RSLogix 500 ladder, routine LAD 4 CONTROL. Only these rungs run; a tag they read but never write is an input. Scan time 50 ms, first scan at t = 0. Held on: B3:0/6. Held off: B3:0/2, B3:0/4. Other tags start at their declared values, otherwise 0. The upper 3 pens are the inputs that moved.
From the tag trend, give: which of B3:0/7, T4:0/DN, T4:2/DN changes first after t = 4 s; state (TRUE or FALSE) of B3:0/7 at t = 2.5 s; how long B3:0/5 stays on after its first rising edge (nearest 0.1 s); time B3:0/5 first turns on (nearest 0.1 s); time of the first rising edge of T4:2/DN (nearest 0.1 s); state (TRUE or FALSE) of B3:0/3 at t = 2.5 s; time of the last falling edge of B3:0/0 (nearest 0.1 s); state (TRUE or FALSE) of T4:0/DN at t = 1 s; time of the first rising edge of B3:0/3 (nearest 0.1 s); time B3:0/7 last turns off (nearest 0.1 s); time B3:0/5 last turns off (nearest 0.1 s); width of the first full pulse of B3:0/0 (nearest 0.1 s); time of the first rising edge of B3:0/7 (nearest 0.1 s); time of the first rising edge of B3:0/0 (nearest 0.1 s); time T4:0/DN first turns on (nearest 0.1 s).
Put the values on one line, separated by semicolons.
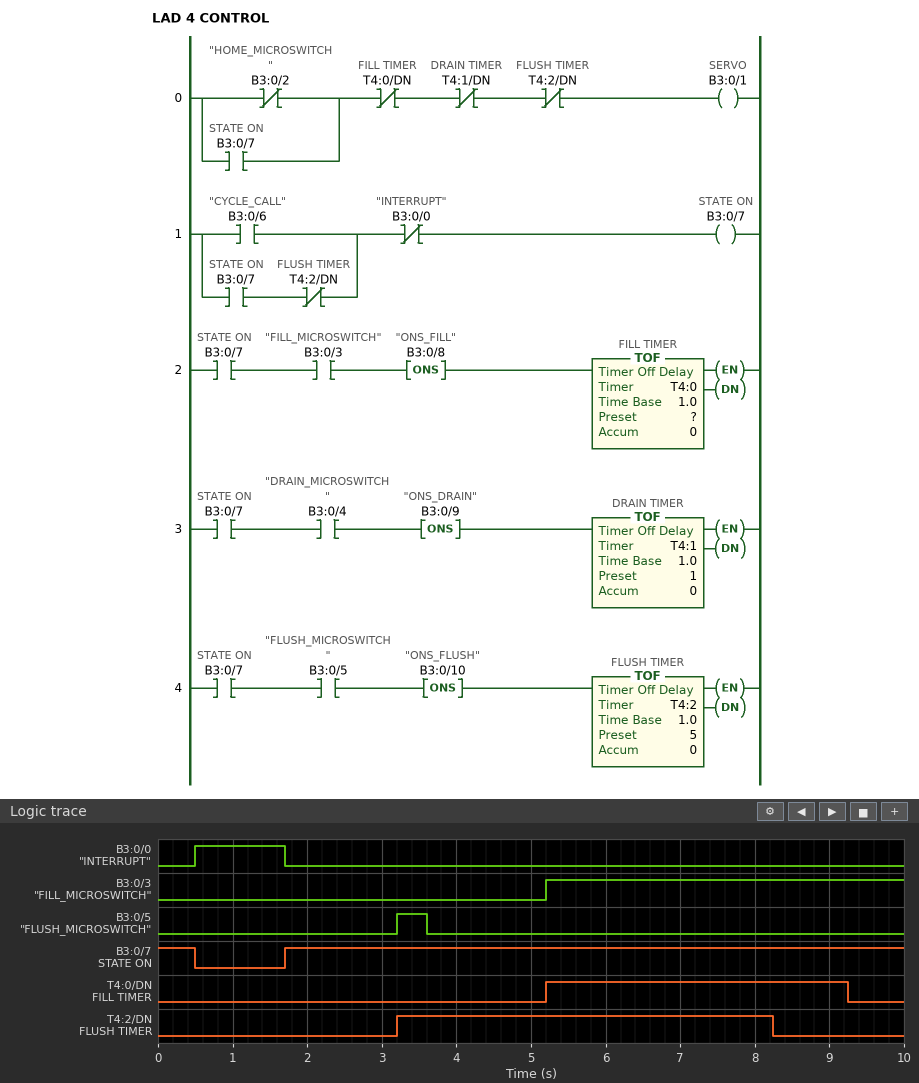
T4:0/DN; TRUE; 0.4 s; 3.2 s; 3.2 s; FALSE; 1.7 s; FALSE; 5.2 s; 0.5 s; 3.6 s; 1.2 s; 1.7 s; 0.5 s; 5.2 s
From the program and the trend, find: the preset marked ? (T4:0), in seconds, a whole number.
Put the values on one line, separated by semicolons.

4 s
